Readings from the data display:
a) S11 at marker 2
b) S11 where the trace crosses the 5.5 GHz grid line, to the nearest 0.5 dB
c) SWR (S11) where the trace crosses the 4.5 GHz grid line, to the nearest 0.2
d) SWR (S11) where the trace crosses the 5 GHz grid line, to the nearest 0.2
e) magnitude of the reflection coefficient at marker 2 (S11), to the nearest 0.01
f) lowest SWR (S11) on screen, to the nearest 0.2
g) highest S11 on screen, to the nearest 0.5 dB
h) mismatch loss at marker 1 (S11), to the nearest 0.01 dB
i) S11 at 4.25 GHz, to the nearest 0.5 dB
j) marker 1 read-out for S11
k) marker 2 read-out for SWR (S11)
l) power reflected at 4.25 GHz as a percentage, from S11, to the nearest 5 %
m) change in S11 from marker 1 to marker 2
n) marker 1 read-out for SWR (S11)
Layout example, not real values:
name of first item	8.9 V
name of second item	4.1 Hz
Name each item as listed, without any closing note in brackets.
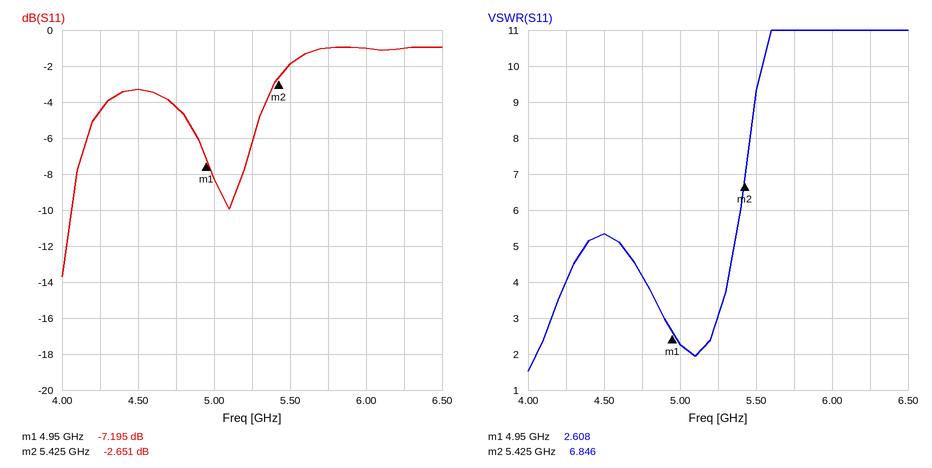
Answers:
S11 at marker 2	-2.651 dB
S11 where the trace crosses the 5.5 GHz grid line, to the nearest 0.5 dB	-2.0 dB
SWR (S11) where the trace crosses the 4.5 GHz grid line, to the nearest 0.2	5.4
SWR (S11) where the trace crosses the 5 GHz grid line, to the nearest 0.2	2.2
magnitude of the reflection coefficient at marker 2 (S11), to the nearest 0.01	0.74
lowest SWR (S11) on screen, to the nearest 0.2	1.6
highest S11 on screen, to the nearest 0.5 dB	-1.0 dB
mismatch loss at marker 1 (S11), to the nearest 0.01 dB	0.92 dB
S11 at 4.25 GHz, to the nearest 0.5 dB	-4.5 dB
marker 1 read-out for S11	-7.195 dB
marker 2 read-out for SWR	6.846
power reflected at 4.25 GHz as a percentage, from S11, to the nearest 5 %	35 %
change in S11 from marker 1 to marker 2	4.544 dB
marker 1 read-out for SWR	2.608
